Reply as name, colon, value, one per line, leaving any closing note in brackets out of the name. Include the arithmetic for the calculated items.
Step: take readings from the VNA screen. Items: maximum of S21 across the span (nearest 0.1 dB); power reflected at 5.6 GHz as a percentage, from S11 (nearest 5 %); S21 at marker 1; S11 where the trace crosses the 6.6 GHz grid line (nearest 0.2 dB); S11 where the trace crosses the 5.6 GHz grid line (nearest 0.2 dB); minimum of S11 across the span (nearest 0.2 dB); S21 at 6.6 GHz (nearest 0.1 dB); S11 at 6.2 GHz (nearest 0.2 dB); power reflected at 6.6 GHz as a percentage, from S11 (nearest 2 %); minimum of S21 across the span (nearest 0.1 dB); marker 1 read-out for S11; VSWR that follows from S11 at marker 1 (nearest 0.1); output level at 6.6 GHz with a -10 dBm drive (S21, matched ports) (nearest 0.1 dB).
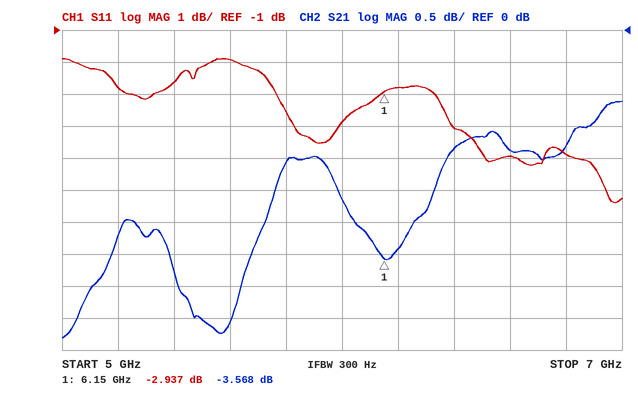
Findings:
maximum of S21 across the span: -1.1 dB
power reflected at 5.6 GHz as a percentage, from S11: 10^(-2/10) ≈ 63.1 %, so 65 % to the nearest 5 %
S21 at marker 1: -3.568 dB
S11 where the trace crosses the 6.6 GHz grid line: -5.0 dB
S11 where the trace crosses the 5.6 GHz grid line: -2.0 dB
minimum of S11 across the span: -6.4 dB
S21 at 6.6 GHz: -1.9 dB
S11 at 6.2 GHz: -2.8 dB
power reflected at 6.6 GHz as a percentage, from S11: 10^(-5/10) ≈ 32 %
minimum of S21 across the span: -4.8 dB
marker 1 read-out for S11: -2.937 dB
VSWR that follows from S11 at marker 1: (1 + 0.7131)/(1 − 0.7131) ≈ 6.0
output level at 6.6 GHz with a -10 dBm drive (S21, matched ports): -10 dBm + (-1.9 dB) = -11.9 dBm
